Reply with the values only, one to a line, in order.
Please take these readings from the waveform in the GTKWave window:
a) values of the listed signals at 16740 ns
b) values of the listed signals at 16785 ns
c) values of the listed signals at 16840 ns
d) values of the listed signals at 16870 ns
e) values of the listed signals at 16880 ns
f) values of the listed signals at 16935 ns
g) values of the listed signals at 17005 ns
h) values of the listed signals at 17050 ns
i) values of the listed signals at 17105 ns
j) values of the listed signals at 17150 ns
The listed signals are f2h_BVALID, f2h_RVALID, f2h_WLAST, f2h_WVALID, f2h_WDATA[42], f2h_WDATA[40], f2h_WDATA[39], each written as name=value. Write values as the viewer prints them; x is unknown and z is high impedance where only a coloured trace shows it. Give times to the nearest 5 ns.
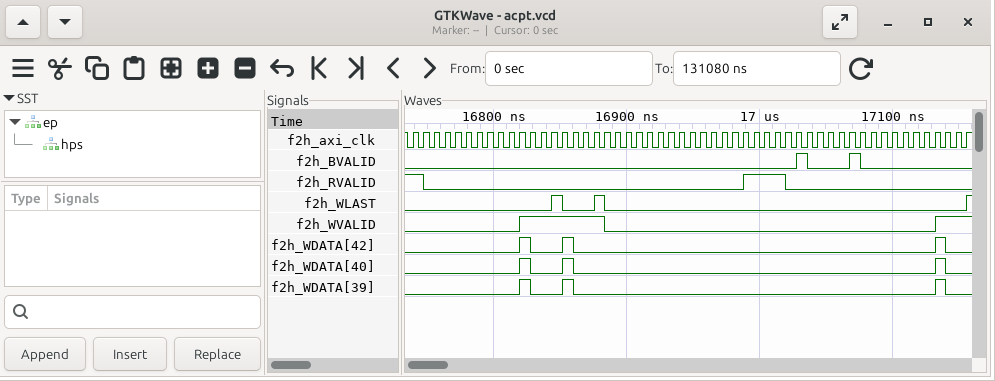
f2h_BVALID=0, f2h_RVALID=1, f2h_WLAST=0, f2h_WVALID=0, f2h_WDATA[42]=0, f2h_WDATA[40]=0, f2h_WDATA[39]=0
f2h_BVALID=0, f2h_RVALID=0, f2h_WLAST=0, f2h_WVALID=0, f2h_WDATA[42]=0, f2h_WDATA[40]=0, f2h_WDATA[39]=0
f2h_BVALID=0, f2h_RVALID=0, f2h_WLAST=0, f2h_WVALID=1, f2h_WDATA[42]=0, f2h_WDATA[40]=0, f2h_WDATA[39]=0
f2h_BVALID=0, f2h_RVALID=0, f2h_WLAST=0, f2h_WVALID=1, f2h_WDATA[42]=0, f2h_WDATA[40]=0, f2h_WDATA[39]=0
f2h_BVALID=0, f2h_RVALID=0, f2h_WLAST=1, f2h_WVALID=1, f2h_WDATA[42]=0, f2h_WDATA[40]=0, f2h_WDATA[39]=0
f2h_BVALID=0, f2h_RVALID=0, f2h_WLAST=0, f2h_WVALID=0, f2h_WDATA[42]=0, f2h_WDATA[40]=0, f2h_WDATA[39]=0
f2h_BVALID=0, f2h_RVALID=1, f2h_WLAST=0, f2h_WVALID=0, f2h_WDATA[42]=0, f2h_WDATA[40]=0, f2h_WDATA[39]=0
f2h_BVALID=0, f2h_RVALID=0, f2h_WLAST=0, f2h_WVALID=0, f2h_WDATA[42]=0, f2h_WDATA[40]=0, f2h_WDATA[39]=0
f2h_BVALID=0, f2h_RVALID=0, f2h_WLAST=0, f2h_WVALID=0, f2h_WDATA[42]=0, f2h_WDATA[40]=0, f2h_WDATA[39]=0
f2h_BVALID=0, f2h_RVALID=0, f2h_WLAST=0, f2h_WVALID=1, f2h_WDATA[42]=0, f2h_WDATA[40]=0, f2h_WDATA[39]=0
